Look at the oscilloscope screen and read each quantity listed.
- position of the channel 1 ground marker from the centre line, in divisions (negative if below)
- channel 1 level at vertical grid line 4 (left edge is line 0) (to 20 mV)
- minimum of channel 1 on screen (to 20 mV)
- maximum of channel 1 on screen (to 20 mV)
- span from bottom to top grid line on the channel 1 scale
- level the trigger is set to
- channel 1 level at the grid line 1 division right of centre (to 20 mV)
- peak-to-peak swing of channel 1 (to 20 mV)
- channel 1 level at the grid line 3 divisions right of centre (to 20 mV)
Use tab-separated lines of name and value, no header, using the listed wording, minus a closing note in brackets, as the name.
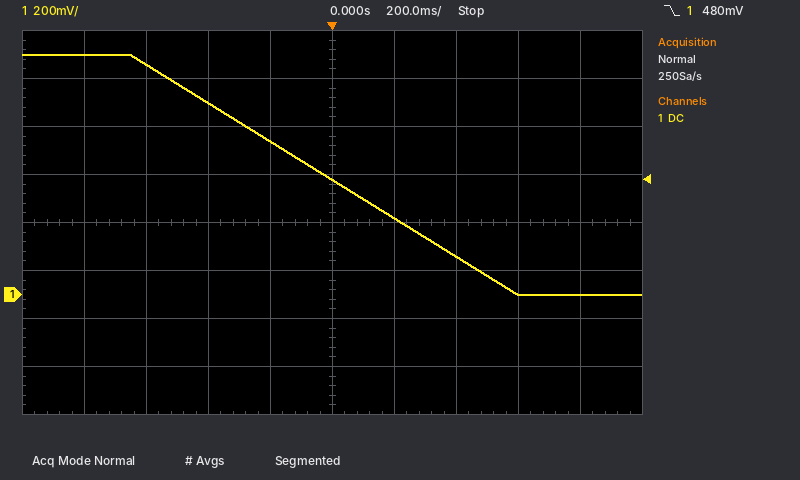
position of the channel 1 ground marker from the centre line, in divisions	-1.5 div
channel 1 level at vertical grid line 4 (left edge is line 0)	640 mV
minimum of channel 1 on screen	0 mV
maximum of channel 1 on screen	1.00 V
span from bottom to top grid line on the channel 1 scale	1.6 V
level the trigger is set to	480 mV
channel 1 level at the grid line 1 division right of centre	320 mV
peak-to-peak swing of channel 1	1.00 V
channel 1 level at the grid line 3 divisions right of centre	0 mV
